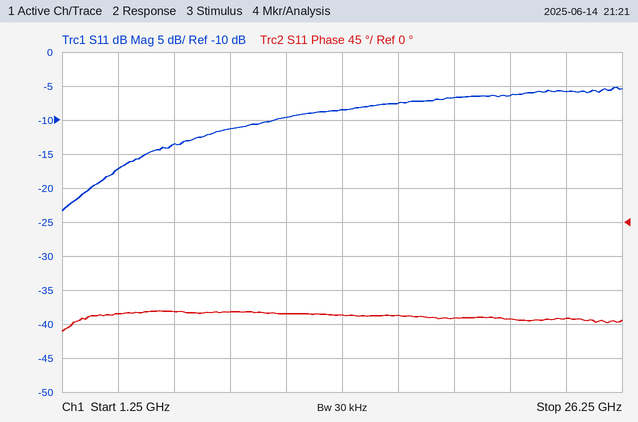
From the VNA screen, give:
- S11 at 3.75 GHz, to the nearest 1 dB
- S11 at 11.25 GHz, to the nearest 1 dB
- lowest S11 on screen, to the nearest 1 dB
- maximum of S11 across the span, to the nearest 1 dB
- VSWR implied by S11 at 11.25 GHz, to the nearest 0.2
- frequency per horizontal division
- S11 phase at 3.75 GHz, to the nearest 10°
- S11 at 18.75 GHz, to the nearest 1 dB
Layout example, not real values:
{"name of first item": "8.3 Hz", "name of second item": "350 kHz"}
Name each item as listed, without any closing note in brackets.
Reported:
{"S11 at 3.75 GHz, to the nearest 1 dB": "-17 dB", "S11 at 11.25 GHz, to the nearest 1 dB": "-10 dB", "lowest S11 on screen, to the nearest 1 dB": "-23 dB", "maximum of S11 across the span, to the nearest 1 dB": "-5 dB", "VSWR implied by S11 at 11.25 GHz, to the nearest 0.2": "2.0", "frequency per horizontal division": "2.5 GHz", "S11 phase at 3.75 GHz, to the nearest 10°": "-120°", "S11 at 18.75 GHz, to the nearest 1 dB": "-7 dB"}
